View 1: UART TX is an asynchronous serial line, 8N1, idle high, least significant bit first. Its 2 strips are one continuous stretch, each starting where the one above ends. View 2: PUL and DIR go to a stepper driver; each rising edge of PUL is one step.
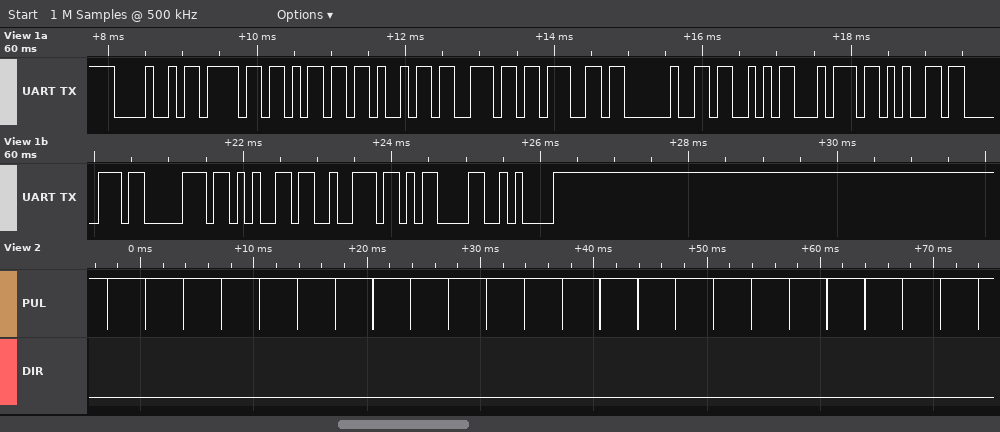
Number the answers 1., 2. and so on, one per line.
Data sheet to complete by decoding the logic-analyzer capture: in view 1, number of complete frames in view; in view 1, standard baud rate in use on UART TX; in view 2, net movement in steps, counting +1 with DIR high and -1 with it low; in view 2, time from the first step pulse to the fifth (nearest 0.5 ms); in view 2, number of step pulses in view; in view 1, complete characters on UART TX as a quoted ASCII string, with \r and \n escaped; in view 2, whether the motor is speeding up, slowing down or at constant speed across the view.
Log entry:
1. 16
2. 9600 baud
3. -24
4. 13.5 ms
5. 24
6. "Homing Stepper\r\n"
7. constant speed
